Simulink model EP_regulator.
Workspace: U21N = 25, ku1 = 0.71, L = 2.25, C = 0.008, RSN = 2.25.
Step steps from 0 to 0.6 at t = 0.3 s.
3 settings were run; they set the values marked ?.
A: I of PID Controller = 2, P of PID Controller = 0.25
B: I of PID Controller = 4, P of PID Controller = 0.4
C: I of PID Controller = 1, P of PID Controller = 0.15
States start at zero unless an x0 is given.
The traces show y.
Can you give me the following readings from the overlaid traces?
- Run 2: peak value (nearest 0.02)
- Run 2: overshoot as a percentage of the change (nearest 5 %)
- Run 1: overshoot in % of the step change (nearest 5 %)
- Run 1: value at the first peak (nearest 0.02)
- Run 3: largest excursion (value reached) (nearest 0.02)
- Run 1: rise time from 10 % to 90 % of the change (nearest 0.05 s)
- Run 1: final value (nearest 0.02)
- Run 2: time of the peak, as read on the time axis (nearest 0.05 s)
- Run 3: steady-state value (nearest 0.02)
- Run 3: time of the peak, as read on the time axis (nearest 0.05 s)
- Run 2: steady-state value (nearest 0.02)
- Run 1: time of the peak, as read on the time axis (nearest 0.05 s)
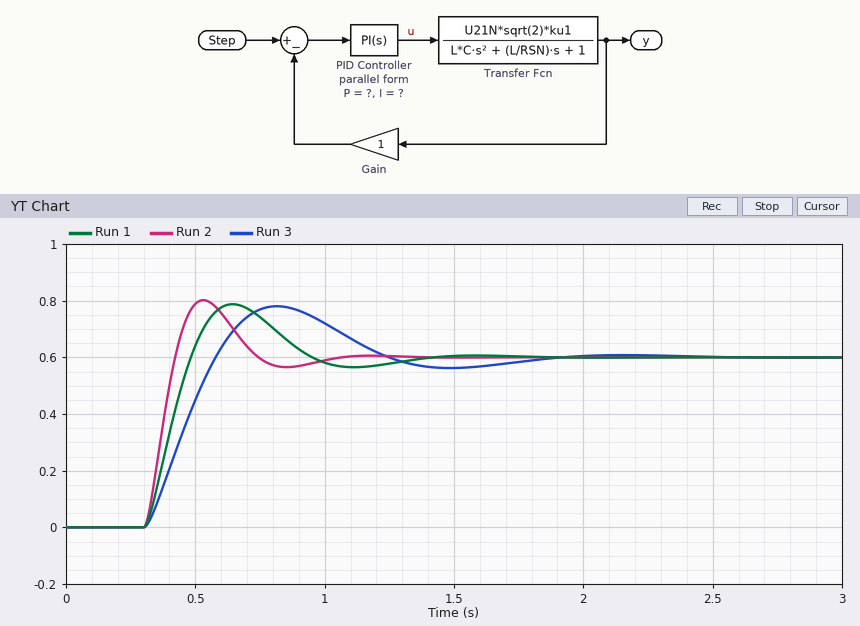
0.80
35 %
30 %
0.78
0.78
0.15 s
0.60
0.55 s
0.60
0.80 s
0.60
0.65 s
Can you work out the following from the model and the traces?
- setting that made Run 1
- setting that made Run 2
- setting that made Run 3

A
B
C
